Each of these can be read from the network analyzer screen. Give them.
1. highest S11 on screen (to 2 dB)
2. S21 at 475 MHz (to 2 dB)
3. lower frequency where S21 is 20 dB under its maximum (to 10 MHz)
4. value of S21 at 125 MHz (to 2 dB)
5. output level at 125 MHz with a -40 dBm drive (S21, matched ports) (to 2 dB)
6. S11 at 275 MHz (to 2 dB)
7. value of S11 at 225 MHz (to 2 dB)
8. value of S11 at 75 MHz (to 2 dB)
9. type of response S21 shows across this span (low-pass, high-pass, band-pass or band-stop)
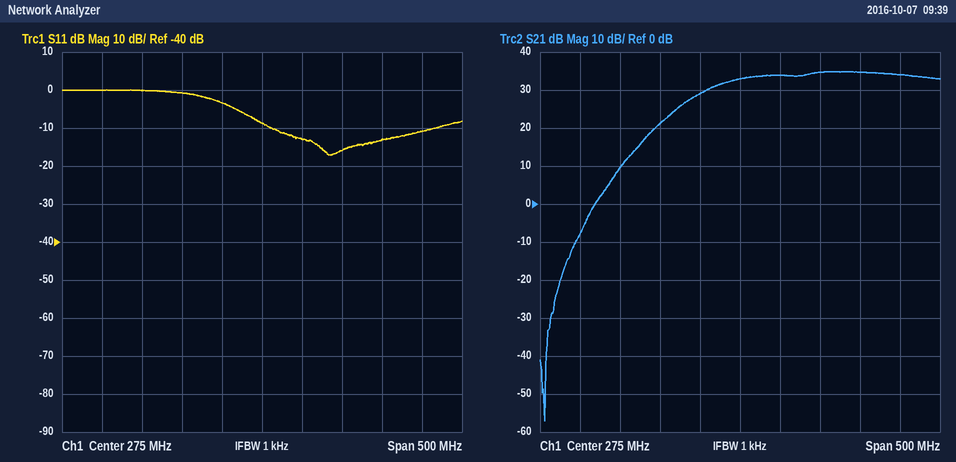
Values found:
0 dB
34 dB
150 MHz
10 dB
-30 dBm
-8 dB
-4 dB
0 dB
high-pass
